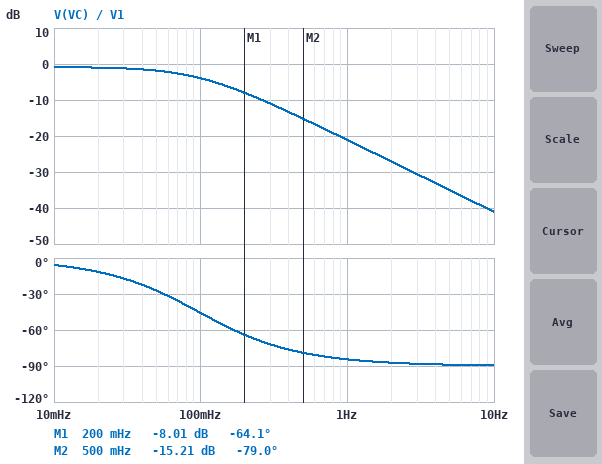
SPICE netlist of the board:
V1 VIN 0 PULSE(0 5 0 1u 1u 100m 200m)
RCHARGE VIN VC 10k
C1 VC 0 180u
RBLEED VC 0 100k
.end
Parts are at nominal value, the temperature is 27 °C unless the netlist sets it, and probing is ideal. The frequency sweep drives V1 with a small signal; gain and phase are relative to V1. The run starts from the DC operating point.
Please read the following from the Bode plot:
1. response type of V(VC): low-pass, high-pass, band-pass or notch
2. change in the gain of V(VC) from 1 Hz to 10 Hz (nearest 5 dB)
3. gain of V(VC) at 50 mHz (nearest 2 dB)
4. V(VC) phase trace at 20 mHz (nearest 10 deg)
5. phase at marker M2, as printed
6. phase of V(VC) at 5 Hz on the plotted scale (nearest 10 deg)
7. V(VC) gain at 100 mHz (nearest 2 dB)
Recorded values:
low-pass
-20 dB
-2 dB
-10 deg
-79.0 deg
-90 deg
-4 dB
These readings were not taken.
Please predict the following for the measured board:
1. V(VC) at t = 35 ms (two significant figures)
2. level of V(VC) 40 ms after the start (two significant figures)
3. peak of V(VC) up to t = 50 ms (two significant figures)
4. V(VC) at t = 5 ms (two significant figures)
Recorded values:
96 mV
110 mV
140 mV
14 mV
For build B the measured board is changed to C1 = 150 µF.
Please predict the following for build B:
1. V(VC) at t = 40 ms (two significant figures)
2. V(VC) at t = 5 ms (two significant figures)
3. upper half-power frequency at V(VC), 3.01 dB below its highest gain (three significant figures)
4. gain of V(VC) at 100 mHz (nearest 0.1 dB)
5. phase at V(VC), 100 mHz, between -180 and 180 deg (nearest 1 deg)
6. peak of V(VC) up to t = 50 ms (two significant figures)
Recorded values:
130 mV
17 mV
117 mHz
-3.2 dB
-41 deg
160 mV
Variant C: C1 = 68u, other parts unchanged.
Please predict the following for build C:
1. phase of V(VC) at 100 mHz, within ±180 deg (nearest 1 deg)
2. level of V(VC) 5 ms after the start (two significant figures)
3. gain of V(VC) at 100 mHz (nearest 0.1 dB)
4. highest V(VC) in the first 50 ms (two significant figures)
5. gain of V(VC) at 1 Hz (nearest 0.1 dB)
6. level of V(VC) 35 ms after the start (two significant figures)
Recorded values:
-21 deg
37 mV
-1.4 dB
350 mV
-12.9 dB
250 mV
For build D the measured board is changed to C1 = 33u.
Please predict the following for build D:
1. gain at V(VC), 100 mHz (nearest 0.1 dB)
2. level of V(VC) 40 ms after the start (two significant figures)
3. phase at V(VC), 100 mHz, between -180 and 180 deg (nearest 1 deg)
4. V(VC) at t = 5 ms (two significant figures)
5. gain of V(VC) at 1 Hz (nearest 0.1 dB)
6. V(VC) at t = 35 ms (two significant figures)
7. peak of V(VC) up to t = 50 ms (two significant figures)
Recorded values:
-1.0 dB
570 mV
-11 deg
75 mV
-7.4 dB
500 mV
700 mV
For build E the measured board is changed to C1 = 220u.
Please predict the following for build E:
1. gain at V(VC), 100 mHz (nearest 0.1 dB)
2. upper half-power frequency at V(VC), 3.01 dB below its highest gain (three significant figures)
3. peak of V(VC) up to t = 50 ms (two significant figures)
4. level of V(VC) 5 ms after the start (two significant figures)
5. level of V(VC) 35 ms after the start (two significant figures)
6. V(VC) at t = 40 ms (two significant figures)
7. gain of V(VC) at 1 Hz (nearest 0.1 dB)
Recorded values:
-4.9 dB
79.6 mHz
110 mV
11 mV
79 mV
90 mV
-22.8 dB
